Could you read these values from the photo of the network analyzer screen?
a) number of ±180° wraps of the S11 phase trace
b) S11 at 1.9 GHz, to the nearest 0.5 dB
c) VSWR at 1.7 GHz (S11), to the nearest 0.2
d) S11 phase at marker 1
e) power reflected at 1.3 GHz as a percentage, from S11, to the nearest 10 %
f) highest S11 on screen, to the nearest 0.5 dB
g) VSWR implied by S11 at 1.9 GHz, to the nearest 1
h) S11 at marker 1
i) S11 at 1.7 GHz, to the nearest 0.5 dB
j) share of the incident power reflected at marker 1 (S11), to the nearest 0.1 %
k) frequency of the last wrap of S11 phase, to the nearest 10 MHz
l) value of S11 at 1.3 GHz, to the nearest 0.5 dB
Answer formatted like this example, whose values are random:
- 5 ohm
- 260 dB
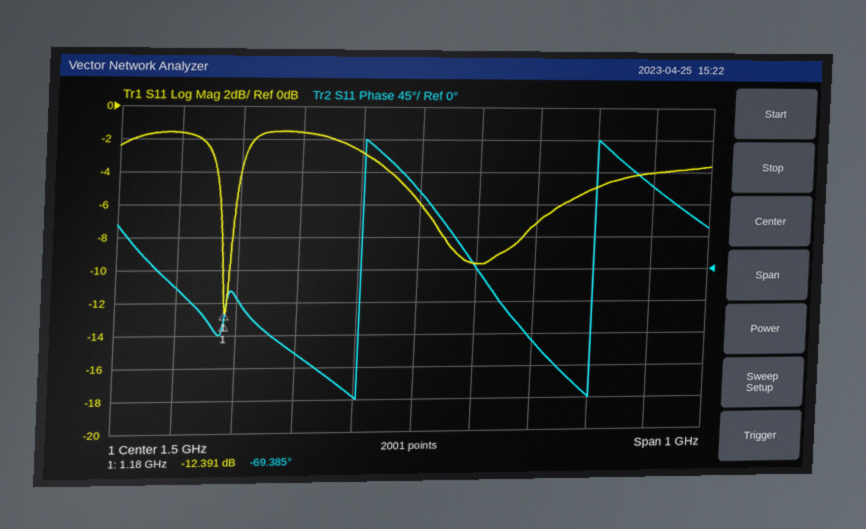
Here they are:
- 2
- -4.0 dB
- 2.6
- -69.385°
- 70 %
- -1.5 dB
- 4
- -12.391 dB
- -7.0 dB
- 5.8 %
- 1.80 GHz
- -1.5 dB
